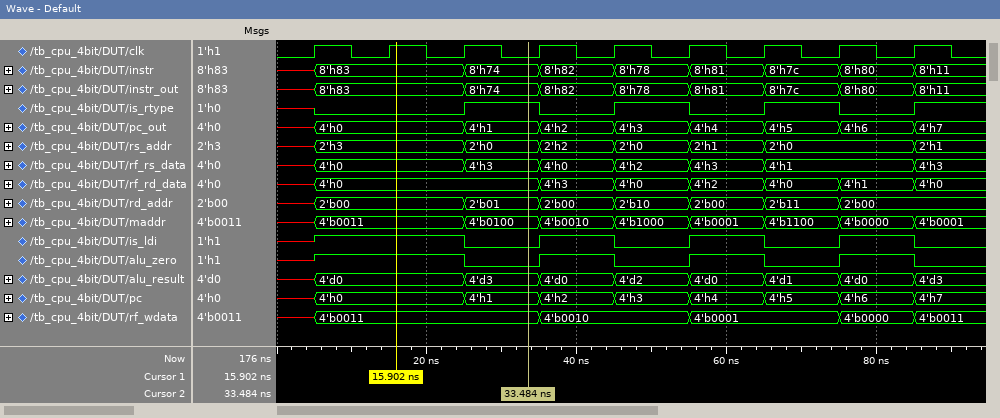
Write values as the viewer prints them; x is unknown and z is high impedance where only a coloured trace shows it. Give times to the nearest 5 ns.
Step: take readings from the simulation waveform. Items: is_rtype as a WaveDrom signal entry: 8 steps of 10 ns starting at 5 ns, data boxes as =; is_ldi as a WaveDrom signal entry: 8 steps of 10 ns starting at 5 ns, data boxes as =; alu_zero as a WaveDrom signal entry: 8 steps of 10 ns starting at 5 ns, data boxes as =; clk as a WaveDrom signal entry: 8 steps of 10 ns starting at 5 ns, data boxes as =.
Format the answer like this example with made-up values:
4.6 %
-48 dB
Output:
{name: 'is_rtype', wave: '0.101010'}
{name: 'is_ldi', wave: '1.010101'}
{name: 'alu_zero', wave: '1.010101'}
{name: 'clk', wave: 'p.......'}
